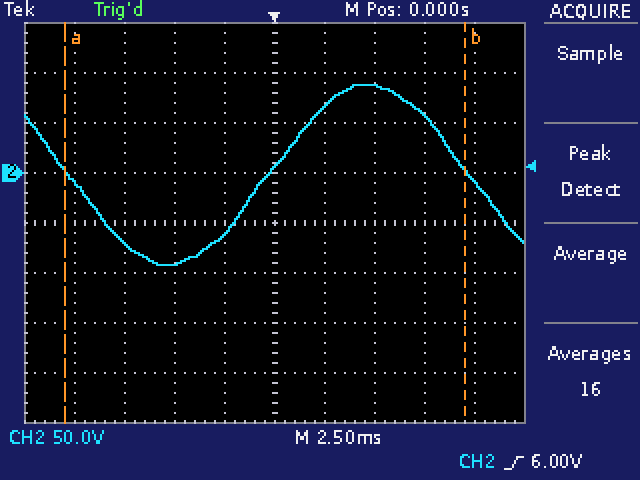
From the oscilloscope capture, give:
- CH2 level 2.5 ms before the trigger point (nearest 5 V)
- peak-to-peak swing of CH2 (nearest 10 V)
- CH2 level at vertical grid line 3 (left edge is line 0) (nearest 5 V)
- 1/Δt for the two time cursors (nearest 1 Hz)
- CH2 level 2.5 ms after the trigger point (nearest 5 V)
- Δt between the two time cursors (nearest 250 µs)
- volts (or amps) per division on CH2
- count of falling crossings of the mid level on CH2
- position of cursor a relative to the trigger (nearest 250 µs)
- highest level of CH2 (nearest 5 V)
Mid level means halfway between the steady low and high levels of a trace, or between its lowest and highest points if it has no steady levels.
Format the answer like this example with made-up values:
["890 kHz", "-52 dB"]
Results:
["-60 V", "180 V", "-90 V", "50 Hz", "65 V", "20.00 ms", "50 V", "2", "-10.50 ms", "90 V"]
